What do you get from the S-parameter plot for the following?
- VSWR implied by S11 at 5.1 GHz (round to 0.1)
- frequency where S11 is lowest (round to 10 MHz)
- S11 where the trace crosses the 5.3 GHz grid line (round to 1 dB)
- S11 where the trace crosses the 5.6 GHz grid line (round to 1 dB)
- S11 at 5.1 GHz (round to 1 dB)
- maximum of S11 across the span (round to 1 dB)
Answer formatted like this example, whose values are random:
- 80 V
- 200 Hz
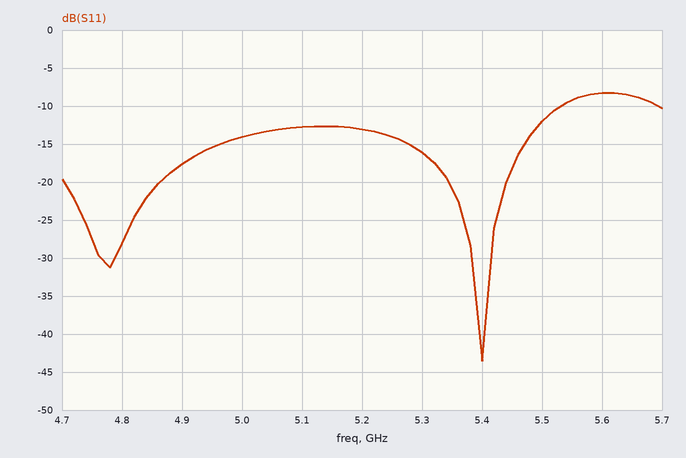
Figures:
- 1.6
- 5.40 GHz
- -16 dB
- -8 dB
- -13 dB
- -8 dB
